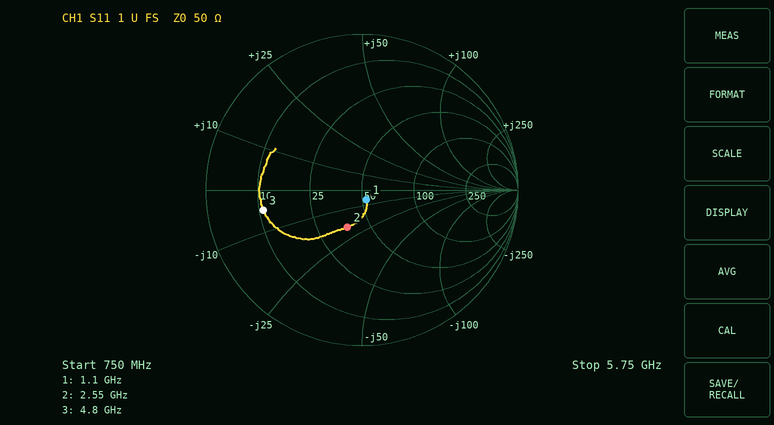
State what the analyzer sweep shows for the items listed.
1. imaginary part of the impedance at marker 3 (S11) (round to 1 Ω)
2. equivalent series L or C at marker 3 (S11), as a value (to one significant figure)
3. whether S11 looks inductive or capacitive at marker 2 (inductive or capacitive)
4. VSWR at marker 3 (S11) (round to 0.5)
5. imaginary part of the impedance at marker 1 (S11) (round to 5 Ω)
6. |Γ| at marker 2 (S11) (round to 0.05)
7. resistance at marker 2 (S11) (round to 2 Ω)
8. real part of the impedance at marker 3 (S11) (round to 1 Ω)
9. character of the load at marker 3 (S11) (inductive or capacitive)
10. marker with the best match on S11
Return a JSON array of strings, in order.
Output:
["-5 Ω", "7 pF", "capacitive", "4.5", "-5 Ω", "0.25", "38 Ω", "11 Ω", "capacitive", "marker 1"]
